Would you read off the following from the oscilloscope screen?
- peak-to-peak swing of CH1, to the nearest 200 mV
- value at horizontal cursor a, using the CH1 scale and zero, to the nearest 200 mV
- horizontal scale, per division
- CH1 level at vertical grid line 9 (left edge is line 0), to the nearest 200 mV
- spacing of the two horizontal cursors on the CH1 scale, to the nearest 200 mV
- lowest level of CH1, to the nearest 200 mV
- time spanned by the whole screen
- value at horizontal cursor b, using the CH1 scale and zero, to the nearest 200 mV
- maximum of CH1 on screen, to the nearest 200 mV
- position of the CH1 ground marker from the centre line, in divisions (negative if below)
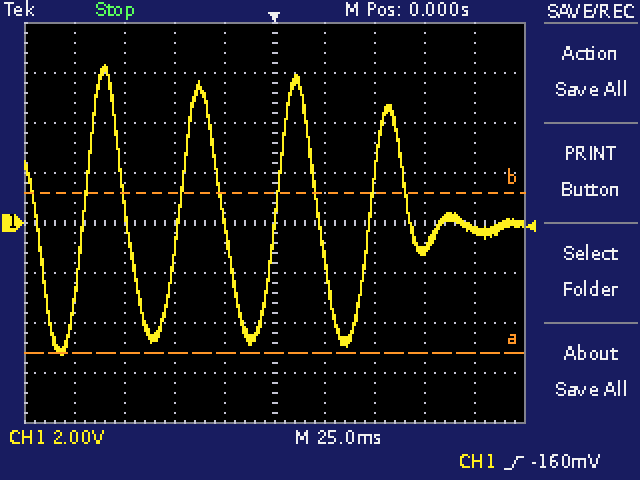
11.6 V
-5.2 V
25 ms
-200 mV
6.4 V
-5.2 V
250 ms
1.2 V
6.4 V
0.0 div
